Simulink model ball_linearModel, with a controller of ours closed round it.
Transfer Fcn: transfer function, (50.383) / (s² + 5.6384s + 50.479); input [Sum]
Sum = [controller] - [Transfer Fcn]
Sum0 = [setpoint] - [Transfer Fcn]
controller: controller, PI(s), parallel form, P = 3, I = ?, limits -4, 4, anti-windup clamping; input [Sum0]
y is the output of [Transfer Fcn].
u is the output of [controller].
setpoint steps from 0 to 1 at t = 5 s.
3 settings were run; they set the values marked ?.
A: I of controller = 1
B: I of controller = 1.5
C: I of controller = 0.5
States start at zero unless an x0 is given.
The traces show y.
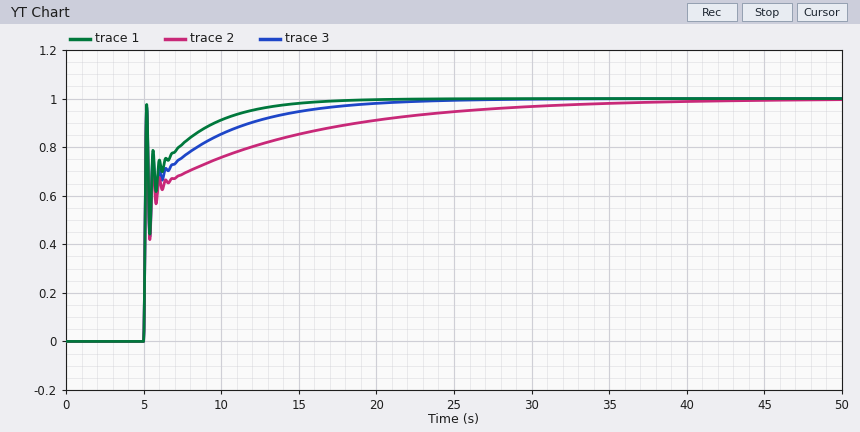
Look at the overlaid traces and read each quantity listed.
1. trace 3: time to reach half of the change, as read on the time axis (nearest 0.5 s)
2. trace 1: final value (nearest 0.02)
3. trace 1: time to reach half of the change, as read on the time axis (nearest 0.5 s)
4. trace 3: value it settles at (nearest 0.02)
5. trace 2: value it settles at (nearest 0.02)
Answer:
5.0 s
1.00
5.0 s
1.00
1.00
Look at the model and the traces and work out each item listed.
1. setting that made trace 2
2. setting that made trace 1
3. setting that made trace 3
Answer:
C
B
A
